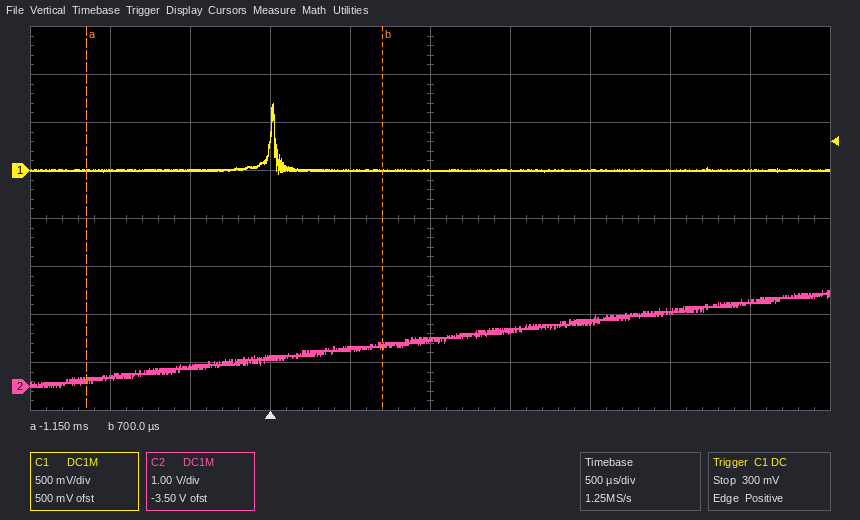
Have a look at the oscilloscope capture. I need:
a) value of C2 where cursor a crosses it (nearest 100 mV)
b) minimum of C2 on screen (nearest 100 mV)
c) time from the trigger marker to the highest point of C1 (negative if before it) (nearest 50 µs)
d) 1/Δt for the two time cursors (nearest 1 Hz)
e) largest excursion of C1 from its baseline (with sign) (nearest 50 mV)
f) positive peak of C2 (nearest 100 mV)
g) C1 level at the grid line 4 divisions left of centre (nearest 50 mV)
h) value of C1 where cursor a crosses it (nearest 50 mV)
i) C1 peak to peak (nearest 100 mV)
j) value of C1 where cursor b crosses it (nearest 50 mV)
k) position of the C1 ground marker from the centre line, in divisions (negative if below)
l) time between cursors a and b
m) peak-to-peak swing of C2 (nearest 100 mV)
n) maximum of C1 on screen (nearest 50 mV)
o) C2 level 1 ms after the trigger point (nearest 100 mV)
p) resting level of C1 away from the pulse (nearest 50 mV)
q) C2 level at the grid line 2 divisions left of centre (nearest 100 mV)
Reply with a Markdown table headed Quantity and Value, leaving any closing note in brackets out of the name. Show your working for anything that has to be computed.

| Quantity | Value |
|---|---|
| value of C2 where cursor a crosses it | 100 mV |
| minimum of C2 on screen | 0.0 V |
| time from the trigger marker to the highest point of C1 (negative if before it) | 0 µs |
| 1/Δt for the two time cursors | 1 / 1.85 ms ≈ 541 Hz |
| largest excursion of C1 from its baseline (with sign) | 700 mV − (0 mV) = +700 mV |
| positive peak of C2 | 2.0 V |
| C1 level at the grid line 4 divisions left of centre | 0 mV |
| value of C1 where cursor a crosses it | 0 mV |
| C1 peak to peak | 700 mV |
| value of C1 where cursor b crosses it | 0 mV |
| position of the C1 ground marker from the centre line, in divisions | +1.0 div |
| time between cursors a and b | 700 µs − (-1.15 ms) = 1.85 ms |
| peak-to-peak swing of C2 | 2.0 V − (0.0 V) = 2.0 V |
| maximum of C1 on screen | 700 mV |
| C2 level 1 ms after the trigger point | 1.0 V |
| resting level of C1 away from the pulse | 0 mV |
| C2 level at the grid line 2 divisions left of centre | 600 mV |
